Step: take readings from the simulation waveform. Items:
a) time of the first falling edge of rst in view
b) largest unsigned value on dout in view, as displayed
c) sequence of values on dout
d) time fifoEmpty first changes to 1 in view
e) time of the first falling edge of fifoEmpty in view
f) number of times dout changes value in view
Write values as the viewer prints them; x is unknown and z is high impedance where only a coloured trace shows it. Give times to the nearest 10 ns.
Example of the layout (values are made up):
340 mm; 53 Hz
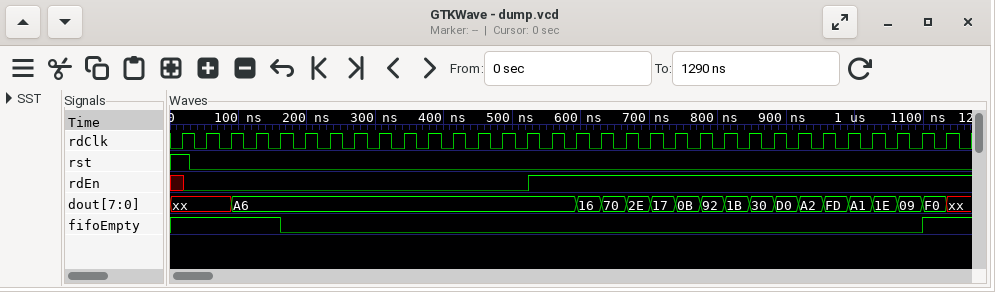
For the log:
30 ns; FD; xx, A6, 16, 70, 2E, 17, 0B, 92, 1B, 30, D0, A2, FD, A1, 1E, 09, F0, xx; 1100 ns; 160 ns; 17
